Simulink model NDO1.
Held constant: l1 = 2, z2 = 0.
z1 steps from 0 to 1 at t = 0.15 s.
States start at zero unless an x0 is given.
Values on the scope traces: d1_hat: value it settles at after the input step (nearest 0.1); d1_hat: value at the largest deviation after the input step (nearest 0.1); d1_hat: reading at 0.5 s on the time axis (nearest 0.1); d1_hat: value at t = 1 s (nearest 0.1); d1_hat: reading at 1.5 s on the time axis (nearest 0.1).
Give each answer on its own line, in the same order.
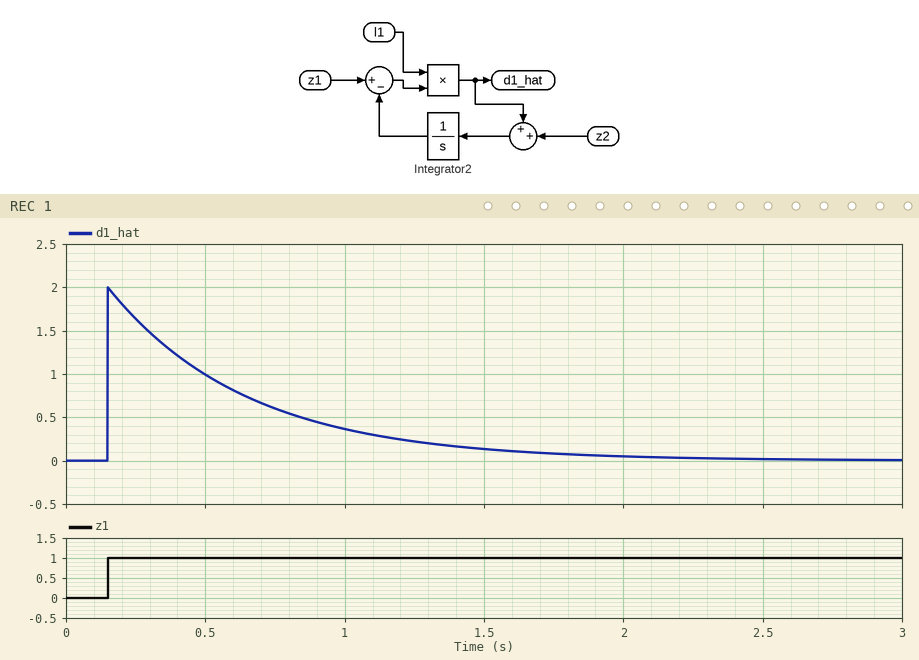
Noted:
0.0
2.0
1.0
0.4
0.1
